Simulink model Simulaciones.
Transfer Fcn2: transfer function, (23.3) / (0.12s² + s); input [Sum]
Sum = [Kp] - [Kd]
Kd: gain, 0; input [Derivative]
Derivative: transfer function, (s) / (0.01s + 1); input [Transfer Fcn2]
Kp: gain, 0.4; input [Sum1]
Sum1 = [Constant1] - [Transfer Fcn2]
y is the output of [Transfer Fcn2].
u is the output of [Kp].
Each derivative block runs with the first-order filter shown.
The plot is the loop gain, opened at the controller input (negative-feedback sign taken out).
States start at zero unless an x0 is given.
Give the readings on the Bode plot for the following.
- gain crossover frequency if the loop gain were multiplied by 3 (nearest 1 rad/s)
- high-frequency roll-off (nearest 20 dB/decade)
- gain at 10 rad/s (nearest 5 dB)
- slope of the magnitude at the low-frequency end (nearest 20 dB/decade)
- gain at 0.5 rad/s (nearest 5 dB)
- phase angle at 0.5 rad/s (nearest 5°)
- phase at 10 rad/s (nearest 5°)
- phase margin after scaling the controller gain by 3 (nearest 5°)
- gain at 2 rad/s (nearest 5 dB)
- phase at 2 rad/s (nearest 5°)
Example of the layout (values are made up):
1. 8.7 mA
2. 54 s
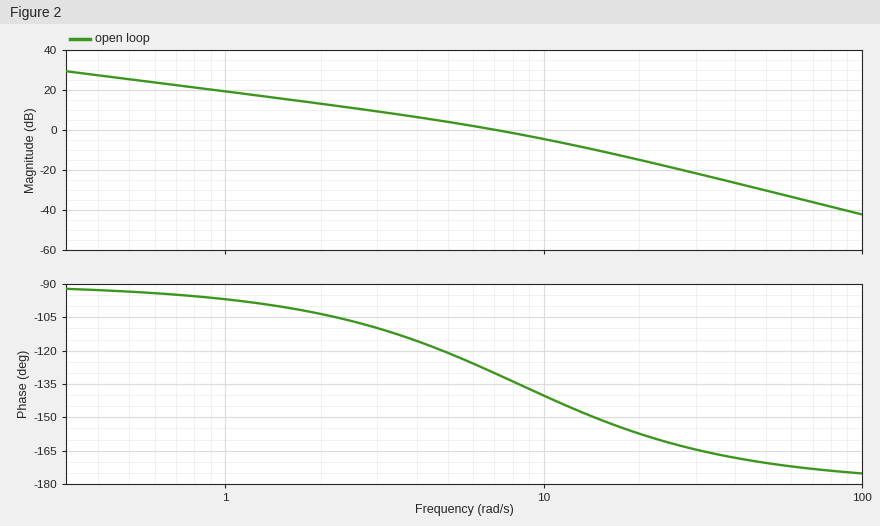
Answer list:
1. 14 rad/s
2. -40 dB/decade
3. -5 dB
4. -20 dB/decade
5. 25 dB
6. -95°
7. -140°
8. 30°
9. 15 dB
10. -105°
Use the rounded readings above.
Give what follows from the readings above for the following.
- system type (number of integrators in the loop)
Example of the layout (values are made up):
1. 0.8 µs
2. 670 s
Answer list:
1. 1
